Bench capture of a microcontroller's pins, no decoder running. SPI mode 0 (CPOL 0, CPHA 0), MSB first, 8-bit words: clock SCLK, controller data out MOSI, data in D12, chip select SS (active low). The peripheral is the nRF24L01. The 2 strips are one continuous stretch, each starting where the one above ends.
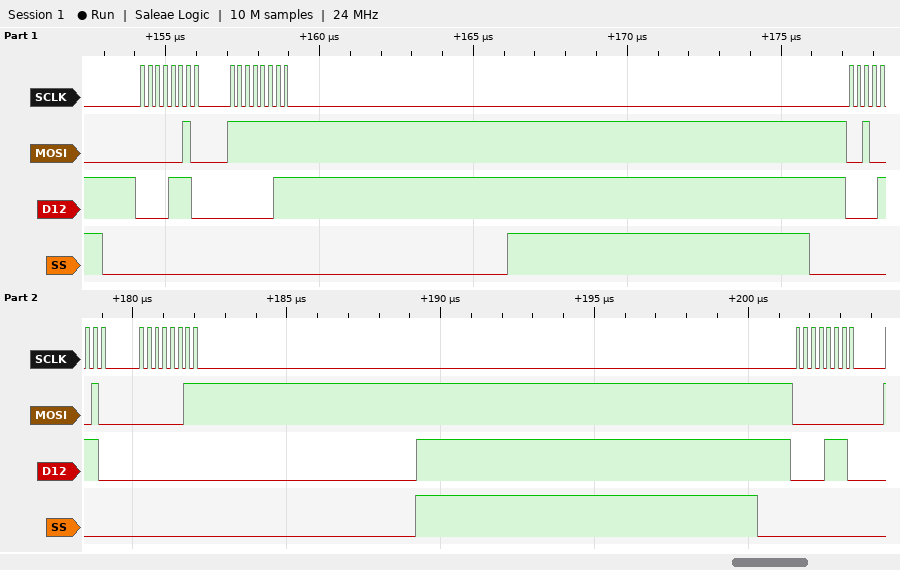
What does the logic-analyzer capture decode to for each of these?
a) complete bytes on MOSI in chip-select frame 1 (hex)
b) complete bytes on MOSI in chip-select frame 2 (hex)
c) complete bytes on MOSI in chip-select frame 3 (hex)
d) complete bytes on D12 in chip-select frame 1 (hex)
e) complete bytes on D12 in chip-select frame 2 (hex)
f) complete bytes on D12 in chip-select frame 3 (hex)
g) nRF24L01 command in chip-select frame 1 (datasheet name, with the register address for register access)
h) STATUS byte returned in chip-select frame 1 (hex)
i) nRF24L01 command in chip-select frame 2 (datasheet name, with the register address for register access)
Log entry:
02 FF
22 03
00
0E 03
0E 00
0E
R_REGISTER 0x02
0x0E
W_REGISTER 0x02
